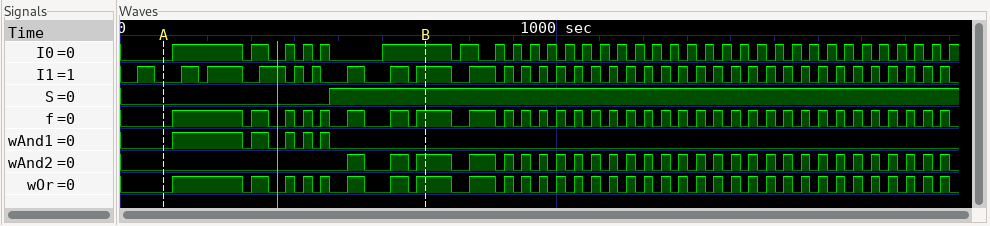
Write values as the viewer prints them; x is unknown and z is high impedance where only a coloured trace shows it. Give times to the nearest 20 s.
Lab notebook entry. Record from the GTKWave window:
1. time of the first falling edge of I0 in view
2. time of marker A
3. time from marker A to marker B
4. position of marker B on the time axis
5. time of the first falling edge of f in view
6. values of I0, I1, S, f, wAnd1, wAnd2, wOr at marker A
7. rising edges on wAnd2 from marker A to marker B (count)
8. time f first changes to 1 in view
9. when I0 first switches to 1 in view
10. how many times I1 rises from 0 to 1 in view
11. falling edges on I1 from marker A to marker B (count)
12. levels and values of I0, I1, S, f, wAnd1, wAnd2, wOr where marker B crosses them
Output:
280 s
100 s
600 s
700 s
280 s
I0=0, I1=0, S=0, f=0, wAnd1=0, wAnd2=0, wOr=0
3
120 s
120 s
36
7
I0=1, I1=1, S=1, f=1, wAnd1=0, wAnd2=1, wOr=1
